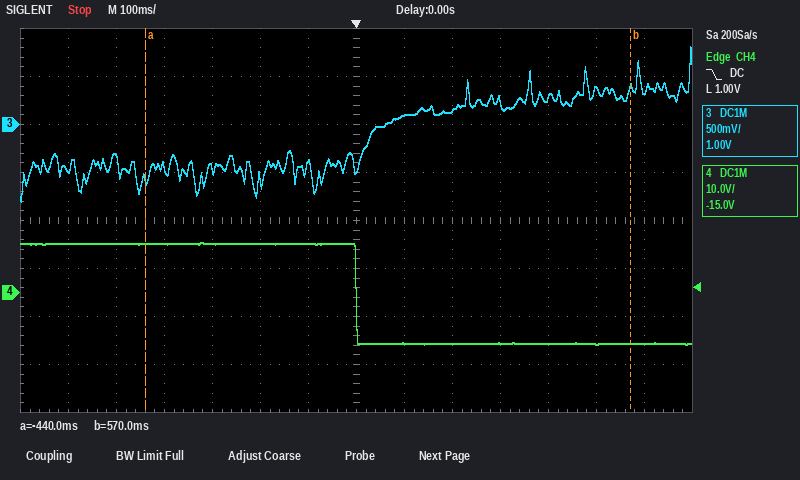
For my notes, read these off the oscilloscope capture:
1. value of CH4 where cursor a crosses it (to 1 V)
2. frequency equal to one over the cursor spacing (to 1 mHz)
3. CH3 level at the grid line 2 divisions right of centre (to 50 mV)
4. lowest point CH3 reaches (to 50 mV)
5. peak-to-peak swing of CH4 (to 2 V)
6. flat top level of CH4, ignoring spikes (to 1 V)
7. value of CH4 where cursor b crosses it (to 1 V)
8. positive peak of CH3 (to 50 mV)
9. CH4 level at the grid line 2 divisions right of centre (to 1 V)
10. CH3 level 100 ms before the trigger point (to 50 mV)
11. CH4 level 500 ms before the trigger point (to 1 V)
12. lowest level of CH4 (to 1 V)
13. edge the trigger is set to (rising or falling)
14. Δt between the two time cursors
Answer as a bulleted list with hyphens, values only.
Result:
- 10 V
- 990 mHz
- 150 mV
- -800 mV
- 22 V
- 10 V
- -11 V
- 800 mV
- -11 V
- -400 mV
- 10 V
- -11 V
- falling
- 1.01 s
